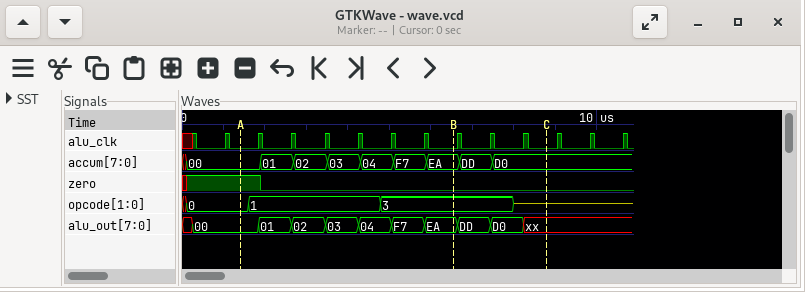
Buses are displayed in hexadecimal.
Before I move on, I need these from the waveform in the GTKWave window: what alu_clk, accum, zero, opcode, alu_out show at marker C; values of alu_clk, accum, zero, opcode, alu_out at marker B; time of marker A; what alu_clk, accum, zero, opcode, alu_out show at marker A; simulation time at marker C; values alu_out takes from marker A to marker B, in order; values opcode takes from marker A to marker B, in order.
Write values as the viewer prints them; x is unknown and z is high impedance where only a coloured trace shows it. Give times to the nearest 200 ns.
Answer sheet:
alu_clk=0, accum=D0, zero=0, opcode=z, alu_out=xx
alu_clk=0, accum=EA, zero=0, opcode=3, alu_out=EA
1400 ns
alu_clk=0, accum=00, zero=1, opcode=0, alu_out=00
8800 ns
00, 01, 02, 03, 04, F7, EA
0, 1, 3
